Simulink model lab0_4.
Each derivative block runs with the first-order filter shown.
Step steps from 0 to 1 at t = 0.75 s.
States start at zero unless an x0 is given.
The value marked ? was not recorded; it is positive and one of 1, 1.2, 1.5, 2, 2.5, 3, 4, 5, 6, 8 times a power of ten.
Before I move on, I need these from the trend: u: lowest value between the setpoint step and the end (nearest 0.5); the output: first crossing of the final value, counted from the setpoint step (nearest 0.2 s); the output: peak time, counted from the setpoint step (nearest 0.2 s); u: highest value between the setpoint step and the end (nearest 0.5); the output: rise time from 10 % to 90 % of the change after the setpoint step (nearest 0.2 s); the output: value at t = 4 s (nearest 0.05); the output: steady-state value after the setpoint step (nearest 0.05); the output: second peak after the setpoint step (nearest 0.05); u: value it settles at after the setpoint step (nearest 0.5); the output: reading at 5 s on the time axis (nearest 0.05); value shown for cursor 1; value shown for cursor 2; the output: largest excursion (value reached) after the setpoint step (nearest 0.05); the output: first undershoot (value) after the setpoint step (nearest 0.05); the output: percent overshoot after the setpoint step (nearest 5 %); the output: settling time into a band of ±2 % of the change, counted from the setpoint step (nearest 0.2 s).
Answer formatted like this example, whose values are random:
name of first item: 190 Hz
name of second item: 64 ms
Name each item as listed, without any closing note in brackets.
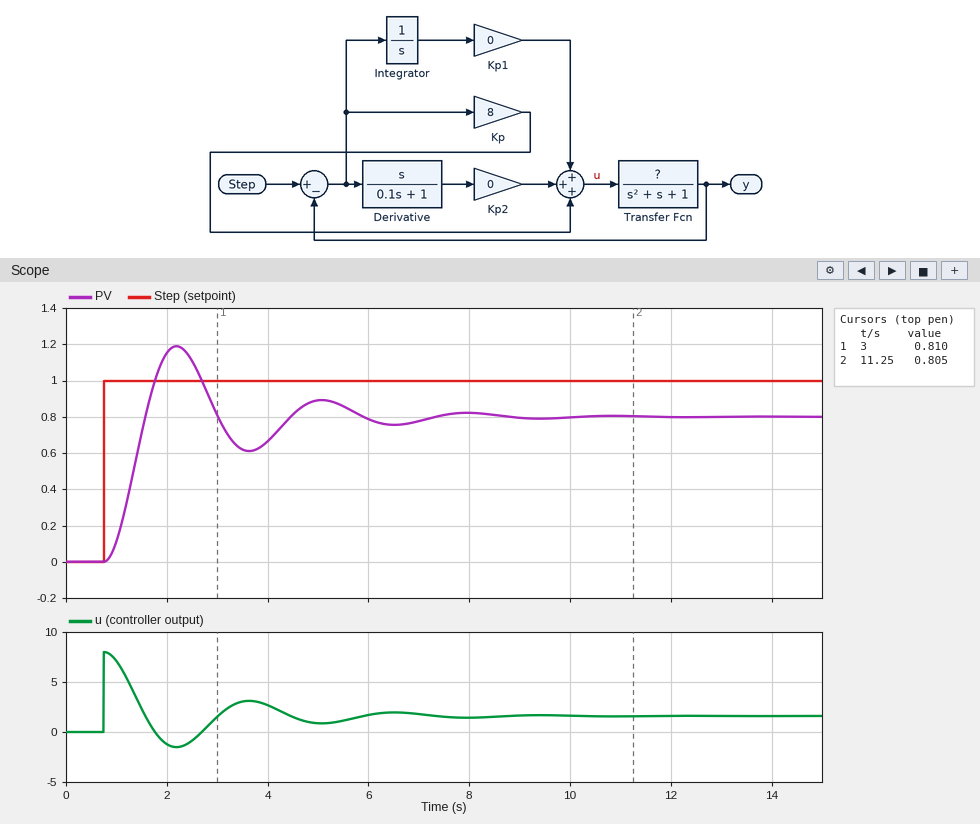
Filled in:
u: lowest value between the setpoint step and the end: -1.5
the output: first crossing of the final value, counted from the setpoint step: 0.8 s
the output: peak time, counted from the setpoint step: 1.4 s
u: highest value between the setpoint step and the end: 8.0
the output: rise time from 10 % to 90 % of the change after the setpoint step: 0.6 s
the output: value at t = 4 s: 0.65
the output: steady-state value after the setpoint step: 0.80
the output: second peak after the setpoint step: 0.90
u: value it settles at after the setpoint step: 1.5
the output: reading at 5 s on the time axis: 0.90
value shown for cursor 1: 0.810
value shown for cursor 2: 0.805
the output: largest excursion (value reached) after the setpoint step: 1.20
the output: first undershoot (value) after the setpoint step: 0.60
the output: percent overshoot after the setpoint step: 50 %
the output: settling time into a band of ±2 % of the change, counted from the setpoint step: 7.6 s
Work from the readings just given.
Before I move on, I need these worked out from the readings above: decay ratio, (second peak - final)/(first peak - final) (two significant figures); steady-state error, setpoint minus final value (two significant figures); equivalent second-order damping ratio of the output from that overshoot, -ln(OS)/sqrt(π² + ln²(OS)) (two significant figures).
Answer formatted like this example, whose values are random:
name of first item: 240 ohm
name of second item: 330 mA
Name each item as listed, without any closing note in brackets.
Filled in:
decay ratio, (second peak - final)/(first peak - final): 0.25
steady-state error, setpoint minus final value: 0.20
equivalent second-order damping ratio of the output from that overshoot, -ln(OS)/sqrt(π² + ln²(OS)): 0.22
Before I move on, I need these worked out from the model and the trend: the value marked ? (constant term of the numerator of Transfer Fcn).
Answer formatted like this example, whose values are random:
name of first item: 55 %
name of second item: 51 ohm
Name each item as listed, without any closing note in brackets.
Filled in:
the value marked ?: 0.5
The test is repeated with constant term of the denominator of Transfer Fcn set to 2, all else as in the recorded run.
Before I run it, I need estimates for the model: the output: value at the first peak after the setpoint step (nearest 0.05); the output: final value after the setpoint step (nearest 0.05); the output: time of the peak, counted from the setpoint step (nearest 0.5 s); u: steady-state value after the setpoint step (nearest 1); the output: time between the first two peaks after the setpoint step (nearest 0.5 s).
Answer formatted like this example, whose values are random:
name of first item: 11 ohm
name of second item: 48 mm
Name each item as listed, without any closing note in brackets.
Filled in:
the output: value at the first peak after the setpoint step: 1.00
the output: final value after the setpoint step: 0.65
the output: time of the peak, counted from the setpoint step: 1.5 s
u: steady-state value after the setpoint step: 3
the output: time between the first two peaks after the setpoint step: 2.5 s
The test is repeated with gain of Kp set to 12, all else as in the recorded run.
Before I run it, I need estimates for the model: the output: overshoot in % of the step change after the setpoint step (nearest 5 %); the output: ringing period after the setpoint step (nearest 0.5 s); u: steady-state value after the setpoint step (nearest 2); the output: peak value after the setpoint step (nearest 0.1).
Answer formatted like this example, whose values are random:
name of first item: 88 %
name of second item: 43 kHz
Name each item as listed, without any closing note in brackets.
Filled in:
the output: overshoot in % of the step change after the setpoint step: 55 %
the output: ringing period after the setpoint step: 2.5 s
u: steady-state value after the setpoint step: 2
the output: peak value after the setpoint step: 1.3
